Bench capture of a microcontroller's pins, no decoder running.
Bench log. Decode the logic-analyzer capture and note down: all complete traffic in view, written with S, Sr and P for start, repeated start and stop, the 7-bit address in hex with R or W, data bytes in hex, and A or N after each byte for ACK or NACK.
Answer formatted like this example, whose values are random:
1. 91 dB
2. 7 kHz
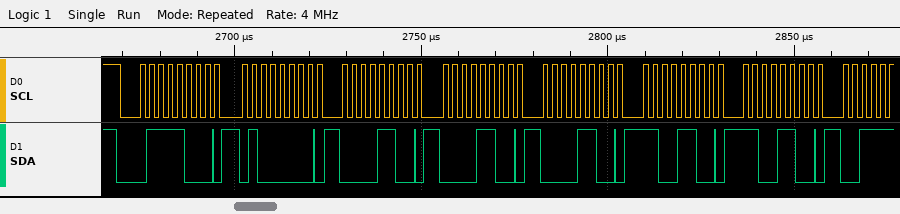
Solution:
1. S 3CW A 40 A 0C A 0C A 0C A CC A CC A
